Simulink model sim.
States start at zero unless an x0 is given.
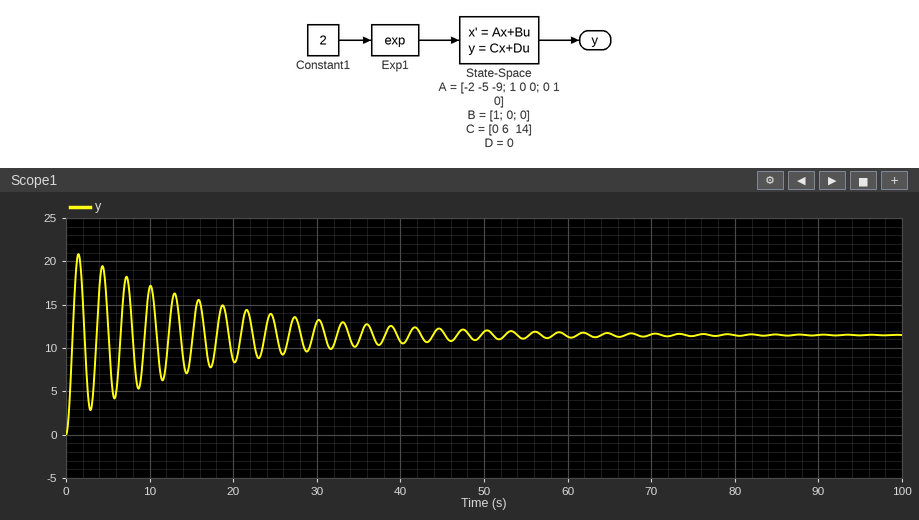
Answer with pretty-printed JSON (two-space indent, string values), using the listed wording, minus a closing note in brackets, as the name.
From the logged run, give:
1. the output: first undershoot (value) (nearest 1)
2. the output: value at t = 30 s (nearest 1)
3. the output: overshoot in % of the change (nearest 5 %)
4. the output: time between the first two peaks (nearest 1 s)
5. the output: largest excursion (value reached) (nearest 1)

{
  "the output: first undershoot (value)": "3",
  "the output: value at t = 30 s": "13",
  "the output: overshoot in % of the change": "80 %",
  "the output: time between the first two peaks": "3 s",
  "the output: largest excursion (value reached)": "21"
}
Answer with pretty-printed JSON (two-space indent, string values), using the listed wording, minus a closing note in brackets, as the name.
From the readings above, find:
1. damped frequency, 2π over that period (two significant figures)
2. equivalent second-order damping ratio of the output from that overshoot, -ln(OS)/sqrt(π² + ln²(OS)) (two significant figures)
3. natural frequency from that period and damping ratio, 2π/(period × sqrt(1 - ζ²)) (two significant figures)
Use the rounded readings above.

{
  "damped frequency, 2π over that period": "2.1 rad/s",
  "equivalent second-order damping ratio of the output from that overshoot, -ln(OS)/sqrt(π² + ln²(OS))": "0.071",
  "natural frequency from that period and damping ratio, 2π/(period × sqrt(1 - ζ²))": "2.1 rad/s"
}
